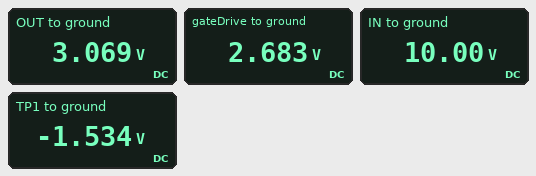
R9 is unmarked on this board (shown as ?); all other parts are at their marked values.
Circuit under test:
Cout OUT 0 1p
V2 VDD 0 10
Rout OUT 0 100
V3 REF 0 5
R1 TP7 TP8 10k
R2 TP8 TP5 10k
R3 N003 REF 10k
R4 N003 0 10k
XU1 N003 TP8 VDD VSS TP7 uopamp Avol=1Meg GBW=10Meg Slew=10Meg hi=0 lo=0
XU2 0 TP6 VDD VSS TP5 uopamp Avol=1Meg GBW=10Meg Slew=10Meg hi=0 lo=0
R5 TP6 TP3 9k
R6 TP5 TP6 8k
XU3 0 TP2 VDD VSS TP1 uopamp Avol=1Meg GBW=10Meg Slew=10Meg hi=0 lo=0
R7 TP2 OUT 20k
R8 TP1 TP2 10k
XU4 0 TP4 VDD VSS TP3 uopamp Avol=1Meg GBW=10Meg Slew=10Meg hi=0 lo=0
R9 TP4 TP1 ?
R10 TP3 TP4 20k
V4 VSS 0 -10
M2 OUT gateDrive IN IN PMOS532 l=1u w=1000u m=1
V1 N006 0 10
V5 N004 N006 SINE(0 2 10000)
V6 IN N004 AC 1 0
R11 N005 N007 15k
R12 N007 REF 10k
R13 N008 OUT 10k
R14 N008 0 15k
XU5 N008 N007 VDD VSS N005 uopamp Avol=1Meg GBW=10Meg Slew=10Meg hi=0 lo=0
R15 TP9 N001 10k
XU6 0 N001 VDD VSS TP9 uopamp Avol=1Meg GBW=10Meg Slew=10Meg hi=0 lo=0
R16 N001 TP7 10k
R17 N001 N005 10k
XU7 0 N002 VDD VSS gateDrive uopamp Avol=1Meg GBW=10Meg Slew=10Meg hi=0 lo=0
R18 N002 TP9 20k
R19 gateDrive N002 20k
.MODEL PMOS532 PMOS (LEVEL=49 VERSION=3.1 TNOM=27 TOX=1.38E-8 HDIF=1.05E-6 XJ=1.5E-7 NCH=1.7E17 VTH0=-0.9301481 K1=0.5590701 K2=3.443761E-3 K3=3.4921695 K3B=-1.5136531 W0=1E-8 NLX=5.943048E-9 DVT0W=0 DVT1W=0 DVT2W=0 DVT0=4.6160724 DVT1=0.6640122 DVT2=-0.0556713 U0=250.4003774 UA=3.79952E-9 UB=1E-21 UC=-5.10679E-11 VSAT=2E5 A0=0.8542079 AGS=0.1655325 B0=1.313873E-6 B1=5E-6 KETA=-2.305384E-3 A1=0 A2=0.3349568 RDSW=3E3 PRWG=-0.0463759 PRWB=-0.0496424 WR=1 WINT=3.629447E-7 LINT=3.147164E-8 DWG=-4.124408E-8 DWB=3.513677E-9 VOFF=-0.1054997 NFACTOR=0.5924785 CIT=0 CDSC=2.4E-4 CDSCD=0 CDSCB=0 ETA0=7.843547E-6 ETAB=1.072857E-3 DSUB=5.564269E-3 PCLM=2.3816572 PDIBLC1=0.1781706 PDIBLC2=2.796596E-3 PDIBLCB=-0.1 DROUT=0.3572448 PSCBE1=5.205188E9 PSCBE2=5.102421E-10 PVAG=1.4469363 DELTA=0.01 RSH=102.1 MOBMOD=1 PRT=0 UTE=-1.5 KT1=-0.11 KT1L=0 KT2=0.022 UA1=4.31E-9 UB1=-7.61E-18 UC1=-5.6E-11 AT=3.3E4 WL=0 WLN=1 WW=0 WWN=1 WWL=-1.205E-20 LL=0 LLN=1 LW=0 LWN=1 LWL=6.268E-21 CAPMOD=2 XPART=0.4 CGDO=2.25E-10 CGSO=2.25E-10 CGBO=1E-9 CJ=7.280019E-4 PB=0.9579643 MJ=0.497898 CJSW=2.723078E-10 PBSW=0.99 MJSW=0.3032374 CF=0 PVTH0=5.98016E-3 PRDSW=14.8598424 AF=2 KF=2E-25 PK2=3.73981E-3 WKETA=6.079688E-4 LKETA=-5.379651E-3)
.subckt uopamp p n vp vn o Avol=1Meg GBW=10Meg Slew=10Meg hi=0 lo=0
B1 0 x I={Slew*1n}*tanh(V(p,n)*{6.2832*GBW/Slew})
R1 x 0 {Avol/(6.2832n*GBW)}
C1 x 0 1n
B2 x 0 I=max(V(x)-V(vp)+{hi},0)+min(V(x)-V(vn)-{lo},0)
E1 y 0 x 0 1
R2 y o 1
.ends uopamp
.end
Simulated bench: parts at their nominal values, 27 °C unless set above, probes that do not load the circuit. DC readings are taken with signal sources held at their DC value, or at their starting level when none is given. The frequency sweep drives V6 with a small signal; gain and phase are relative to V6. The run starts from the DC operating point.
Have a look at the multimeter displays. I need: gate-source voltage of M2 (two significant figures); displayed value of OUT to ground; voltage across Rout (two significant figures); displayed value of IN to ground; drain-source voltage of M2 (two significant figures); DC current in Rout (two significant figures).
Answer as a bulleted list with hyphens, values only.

- -7.3 V
- 3.069 V
- 3.1 V
- 10.00 V
- -6.9 V
- 31 mA
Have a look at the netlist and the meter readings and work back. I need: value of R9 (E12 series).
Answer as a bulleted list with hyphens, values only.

- 47 kΩ
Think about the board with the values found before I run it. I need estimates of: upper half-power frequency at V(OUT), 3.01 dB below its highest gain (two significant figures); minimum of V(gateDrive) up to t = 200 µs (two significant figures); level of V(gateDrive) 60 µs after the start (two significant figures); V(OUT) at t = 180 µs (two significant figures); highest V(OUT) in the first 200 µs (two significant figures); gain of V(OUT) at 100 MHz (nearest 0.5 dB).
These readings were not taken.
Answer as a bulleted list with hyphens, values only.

- 690 MHz
- 1.6 V
- 2.1 V
- 2.5 V
- 3.7 V
- -9.5 dB
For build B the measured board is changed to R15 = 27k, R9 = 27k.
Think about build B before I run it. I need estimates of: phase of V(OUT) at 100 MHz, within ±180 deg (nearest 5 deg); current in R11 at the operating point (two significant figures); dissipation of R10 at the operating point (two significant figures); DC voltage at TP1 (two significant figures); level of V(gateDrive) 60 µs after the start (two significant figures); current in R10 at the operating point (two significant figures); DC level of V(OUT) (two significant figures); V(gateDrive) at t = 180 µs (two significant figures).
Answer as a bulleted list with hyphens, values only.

- -5 deg
- 360 µA
- 38 µW
- -1.2 V
- 4.0 V
- 44 µA
- 2.4 V
- 3.4 V
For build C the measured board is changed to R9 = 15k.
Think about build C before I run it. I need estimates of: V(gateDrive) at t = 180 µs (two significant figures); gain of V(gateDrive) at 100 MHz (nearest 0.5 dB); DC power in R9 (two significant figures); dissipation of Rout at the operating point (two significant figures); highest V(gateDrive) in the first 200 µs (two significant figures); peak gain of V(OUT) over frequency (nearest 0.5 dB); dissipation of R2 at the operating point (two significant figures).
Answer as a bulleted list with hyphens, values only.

- 2.5 V
- -59.0 dB
- 150 µW
- 88 mW
- 4.9 V
- -7.0 dB
- 1.8 mW
